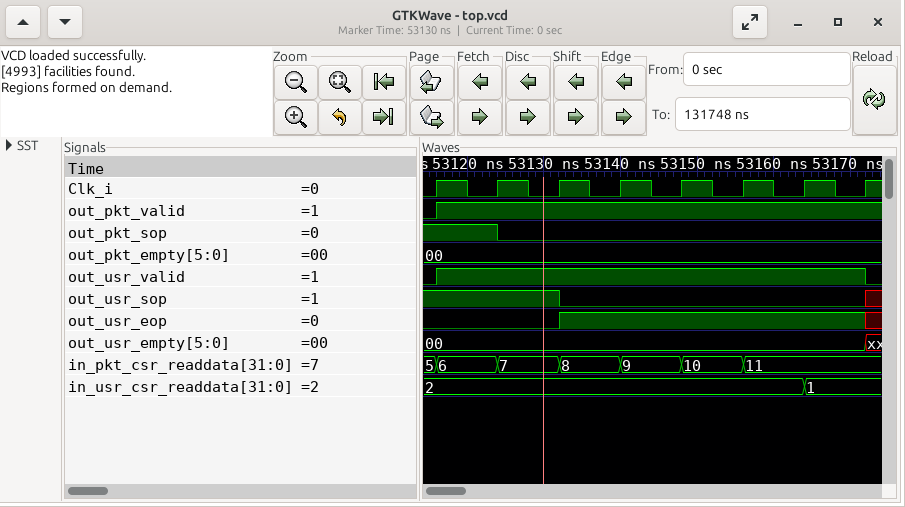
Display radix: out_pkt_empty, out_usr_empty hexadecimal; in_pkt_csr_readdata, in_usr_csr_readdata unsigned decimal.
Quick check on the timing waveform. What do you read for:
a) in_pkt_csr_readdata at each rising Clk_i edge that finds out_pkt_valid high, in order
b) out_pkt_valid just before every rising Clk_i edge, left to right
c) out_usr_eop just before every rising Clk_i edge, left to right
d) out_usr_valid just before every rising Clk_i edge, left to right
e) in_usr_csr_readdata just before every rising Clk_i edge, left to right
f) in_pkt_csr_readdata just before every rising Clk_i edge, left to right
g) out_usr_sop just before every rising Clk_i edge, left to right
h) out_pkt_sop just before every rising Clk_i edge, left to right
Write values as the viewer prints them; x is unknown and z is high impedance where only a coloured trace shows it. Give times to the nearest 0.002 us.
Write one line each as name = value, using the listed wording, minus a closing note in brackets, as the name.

in_pkt_csr_readdata at each rising Clk_i edge that finds out_pkt_valid high, in order = 6, 7, 8, 9, 10, 11, 11
out_pkt_valid just before every rising Clk_i edge, left to right = 0 1 1 1 1 1 1 1
out_usr_eop just before every rising Clk_i edge, left to right = 0 0 0 1 1 1 1 1
out_usr_valid just before every rising Clk_i edge, left to right = 0 1 1 1 1 1 1 1
in_usr_csr_readdata just before every rising Clk_i edge, left to right = 2, 2, 2, 2, 2, 2, 2, 1
in_pkt_csr_readdata just before every rising Clk_i edge, left to right = 5, 6, 7, 8, 9, 10, 11, 11
out_usr_sop just before every rising Clk_i edge, left to right = 1 1 1 0 0 0 0 0
out_pkt_sop just before every rising Clk_i edge, left to right = 1 1 0 0 0 0 0 0
